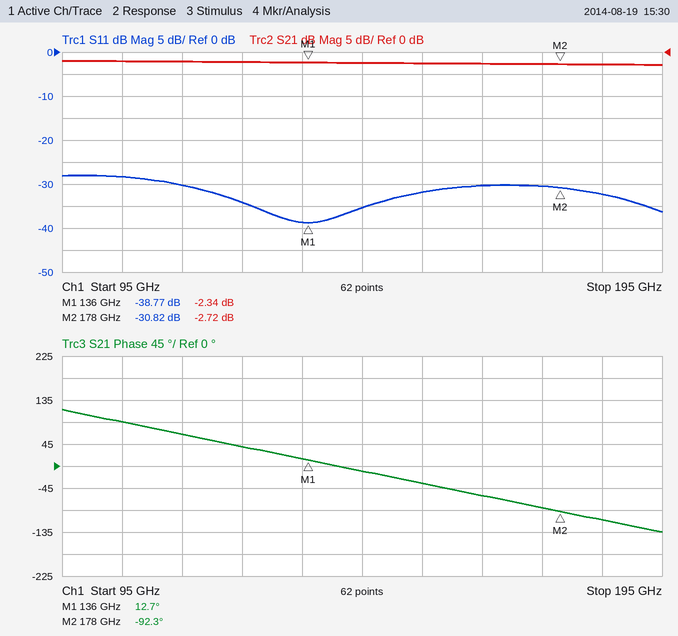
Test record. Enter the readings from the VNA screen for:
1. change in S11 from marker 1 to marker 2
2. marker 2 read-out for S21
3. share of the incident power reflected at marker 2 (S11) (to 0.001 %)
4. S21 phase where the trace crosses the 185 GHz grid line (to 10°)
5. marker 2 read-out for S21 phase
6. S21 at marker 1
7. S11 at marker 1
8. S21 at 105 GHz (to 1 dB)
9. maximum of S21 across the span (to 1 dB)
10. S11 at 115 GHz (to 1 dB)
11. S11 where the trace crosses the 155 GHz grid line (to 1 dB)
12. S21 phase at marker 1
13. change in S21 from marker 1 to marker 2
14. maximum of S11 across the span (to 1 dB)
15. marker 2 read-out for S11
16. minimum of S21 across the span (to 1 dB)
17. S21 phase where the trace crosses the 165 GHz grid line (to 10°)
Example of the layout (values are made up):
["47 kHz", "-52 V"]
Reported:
["7.95 dB", "-2.72 dB", "0.083 %", "-110°", "-92.3°", "-2.34 dB", "-38.77 dB", "-2 dB", "-2 dB", "-30 dB", "-32 dB", "12.7°", "-0.38 dB", "-28 dB", "-30.82 dB", "-3 dB", "-60°"]
